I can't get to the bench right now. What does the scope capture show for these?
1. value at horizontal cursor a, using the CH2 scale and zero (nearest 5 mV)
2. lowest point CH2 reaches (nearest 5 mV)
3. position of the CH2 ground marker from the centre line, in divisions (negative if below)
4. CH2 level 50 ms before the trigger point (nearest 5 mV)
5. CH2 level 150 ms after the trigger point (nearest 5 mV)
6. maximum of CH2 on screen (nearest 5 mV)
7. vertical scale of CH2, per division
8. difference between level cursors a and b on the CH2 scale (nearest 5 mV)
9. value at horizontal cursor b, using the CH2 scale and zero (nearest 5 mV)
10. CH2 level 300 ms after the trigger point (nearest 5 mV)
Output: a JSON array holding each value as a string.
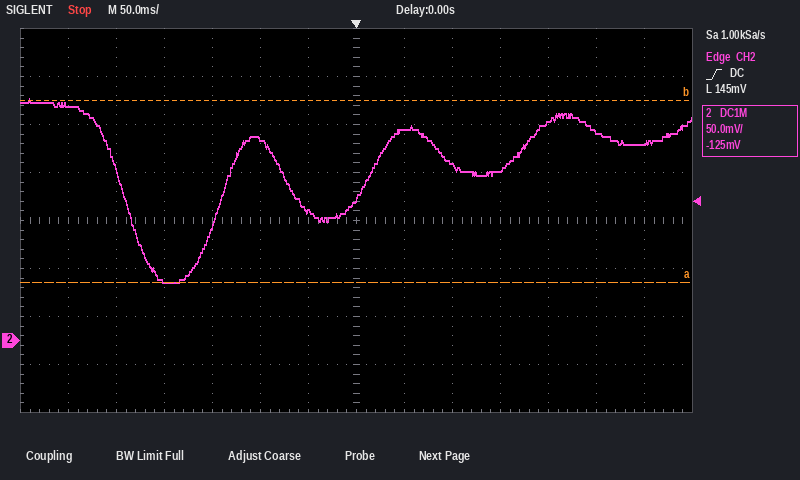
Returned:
["60 mV", "60 mV", "-2.5 div", "135 mV", "175 mV", "250 mV", "50 mV", "190 mV", "250 mV", "205 mV"]
